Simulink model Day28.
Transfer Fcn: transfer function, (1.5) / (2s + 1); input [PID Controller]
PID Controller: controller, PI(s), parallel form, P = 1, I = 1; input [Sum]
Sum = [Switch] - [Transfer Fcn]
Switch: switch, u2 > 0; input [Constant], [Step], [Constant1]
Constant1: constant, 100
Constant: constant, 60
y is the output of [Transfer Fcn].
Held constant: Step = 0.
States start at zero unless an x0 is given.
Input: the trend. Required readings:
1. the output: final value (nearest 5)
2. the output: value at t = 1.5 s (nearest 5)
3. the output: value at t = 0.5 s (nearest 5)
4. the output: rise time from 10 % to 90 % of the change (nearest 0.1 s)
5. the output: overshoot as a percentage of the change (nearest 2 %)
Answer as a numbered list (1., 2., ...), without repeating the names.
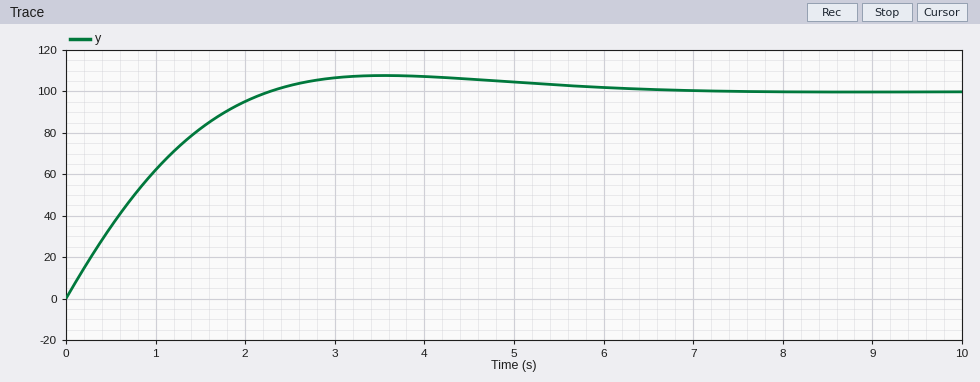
1. 100
2. 80
3. 35
4. 1.6 s
5. 8 %
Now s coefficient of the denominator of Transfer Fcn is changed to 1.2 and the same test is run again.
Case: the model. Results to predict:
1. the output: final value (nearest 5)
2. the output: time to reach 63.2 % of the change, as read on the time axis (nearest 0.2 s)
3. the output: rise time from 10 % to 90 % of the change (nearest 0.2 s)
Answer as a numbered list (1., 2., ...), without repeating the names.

1. 100
2. 0.8 s
3. 1.4 s
